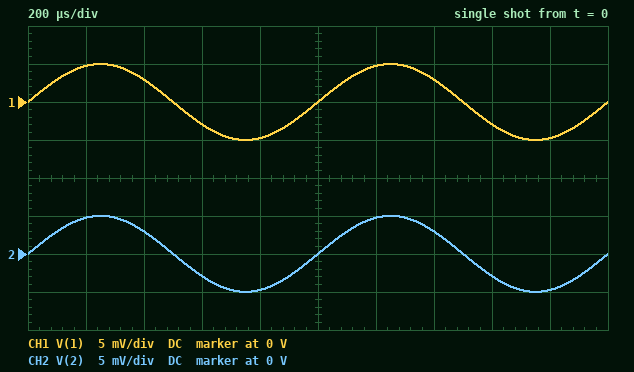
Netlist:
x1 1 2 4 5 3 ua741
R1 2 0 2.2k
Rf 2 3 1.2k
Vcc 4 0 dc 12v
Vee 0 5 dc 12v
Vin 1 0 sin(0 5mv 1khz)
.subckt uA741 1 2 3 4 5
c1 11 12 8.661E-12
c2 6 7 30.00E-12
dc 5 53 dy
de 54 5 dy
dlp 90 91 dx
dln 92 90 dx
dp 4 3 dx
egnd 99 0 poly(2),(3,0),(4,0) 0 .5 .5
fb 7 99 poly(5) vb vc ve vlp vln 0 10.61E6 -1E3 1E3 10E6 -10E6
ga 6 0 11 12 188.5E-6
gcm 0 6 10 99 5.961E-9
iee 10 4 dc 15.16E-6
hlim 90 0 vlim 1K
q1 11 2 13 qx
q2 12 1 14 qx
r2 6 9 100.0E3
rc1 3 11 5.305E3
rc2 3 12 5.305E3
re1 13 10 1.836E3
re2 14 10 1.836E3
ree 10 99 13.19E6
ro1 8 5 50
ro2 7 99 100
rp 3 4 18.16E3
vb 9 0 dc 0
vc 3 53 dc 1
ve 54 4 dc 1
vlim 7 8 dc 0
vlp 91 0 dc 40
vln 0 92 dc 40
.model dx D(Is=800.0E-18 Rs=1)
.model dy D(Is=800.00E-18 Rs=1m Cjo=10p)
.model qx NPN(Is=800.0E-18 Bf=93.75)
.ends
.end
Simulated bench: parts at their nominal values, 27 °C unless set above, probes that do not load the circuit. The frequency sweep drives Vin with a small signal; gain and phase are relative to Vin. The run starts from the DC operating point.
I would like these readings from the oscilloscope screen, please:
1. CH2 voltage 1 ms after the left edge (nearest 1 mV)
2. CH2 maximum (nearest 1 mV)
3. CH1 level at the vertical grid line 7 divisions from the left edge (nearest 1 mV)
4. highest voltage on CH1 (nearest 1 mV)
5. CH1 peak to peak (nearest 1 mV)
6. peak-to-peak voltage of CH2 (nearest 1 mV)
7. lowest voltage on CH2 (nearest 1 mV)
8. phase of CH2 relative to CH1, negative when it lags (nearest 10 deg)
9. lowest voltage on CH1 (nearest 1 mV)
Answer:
0 V
5 mV
3 mV
5 mV
10 mV
10 mV
-5 mV
0 deg
-5 mV
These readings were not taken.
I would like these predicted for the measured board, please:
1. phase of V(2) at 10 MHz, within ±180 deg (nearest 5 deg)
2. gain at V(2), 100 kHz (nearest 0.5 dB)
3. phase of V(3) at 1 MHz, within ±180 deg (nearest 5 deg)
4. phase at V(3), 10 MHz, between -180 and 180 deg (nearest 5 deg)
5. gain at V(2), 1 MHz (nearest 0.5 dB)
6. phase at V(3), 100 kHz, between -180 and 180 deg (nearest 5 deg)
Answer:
-170 deg
0 dB
-85 deg
-170 deg
-4.0 dB
-10 deg
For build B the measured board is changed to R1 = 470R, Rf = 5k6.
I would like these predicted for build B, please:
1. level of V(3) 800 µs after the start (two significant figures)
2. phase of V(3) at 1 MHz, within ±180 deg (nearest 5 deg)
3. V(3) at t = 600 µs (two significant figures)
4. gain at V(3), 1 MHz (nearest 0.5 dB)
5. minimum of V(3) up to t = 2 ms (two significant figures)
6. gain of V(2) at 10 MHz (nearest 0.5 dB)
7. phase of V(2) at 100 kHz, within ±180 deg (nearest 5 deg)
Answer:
-61 mV
-115 deg
-37 mV
-1.0 dB
-64 mV
-61.0 dB
-55 deg
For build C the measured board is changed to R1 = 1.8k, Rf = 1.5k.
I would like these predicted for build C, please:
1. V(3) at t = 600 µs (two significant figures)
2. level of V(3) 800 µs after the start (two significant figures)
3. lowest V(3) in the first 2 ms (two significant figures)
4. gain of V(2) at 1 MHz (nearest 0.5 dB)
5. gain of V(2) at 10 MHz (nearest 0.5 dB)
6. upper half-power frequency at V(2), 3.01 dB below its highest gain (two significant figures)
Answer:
-5.2 mV
-8.6 mV
-9.0 mV
-5.5 dB
-41.5 dB
720 kHz
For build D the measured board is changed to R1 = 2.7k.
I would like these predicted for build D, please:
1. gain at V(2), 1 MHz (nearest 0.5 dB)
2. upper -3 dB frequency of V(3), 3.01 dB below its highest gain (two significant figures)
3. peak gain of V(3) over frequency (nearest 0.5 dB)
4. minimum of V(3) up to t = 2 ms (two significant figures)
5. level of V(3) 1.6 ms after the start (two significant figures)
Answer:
-3.5 dB
950 kHz
3.0 dB
-7.1 mV
-4.1 mV
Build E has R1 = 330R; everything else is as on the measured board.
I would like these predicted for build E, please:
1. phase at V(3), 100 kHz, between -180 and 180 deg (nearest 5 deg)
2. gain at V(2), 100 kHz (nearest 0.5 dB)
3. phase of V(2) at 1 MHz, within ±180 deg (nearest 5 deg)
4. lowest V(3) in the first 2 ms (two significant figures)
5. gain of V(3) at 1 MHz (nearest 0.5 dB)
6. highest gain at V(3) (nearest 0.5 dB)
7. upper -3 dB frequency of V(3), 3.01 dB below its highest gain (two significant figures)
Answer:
-25 deg
-0.5 dB
-110 deg
-23 mV
-1.0 dB
13.5 dB
240 kHz
